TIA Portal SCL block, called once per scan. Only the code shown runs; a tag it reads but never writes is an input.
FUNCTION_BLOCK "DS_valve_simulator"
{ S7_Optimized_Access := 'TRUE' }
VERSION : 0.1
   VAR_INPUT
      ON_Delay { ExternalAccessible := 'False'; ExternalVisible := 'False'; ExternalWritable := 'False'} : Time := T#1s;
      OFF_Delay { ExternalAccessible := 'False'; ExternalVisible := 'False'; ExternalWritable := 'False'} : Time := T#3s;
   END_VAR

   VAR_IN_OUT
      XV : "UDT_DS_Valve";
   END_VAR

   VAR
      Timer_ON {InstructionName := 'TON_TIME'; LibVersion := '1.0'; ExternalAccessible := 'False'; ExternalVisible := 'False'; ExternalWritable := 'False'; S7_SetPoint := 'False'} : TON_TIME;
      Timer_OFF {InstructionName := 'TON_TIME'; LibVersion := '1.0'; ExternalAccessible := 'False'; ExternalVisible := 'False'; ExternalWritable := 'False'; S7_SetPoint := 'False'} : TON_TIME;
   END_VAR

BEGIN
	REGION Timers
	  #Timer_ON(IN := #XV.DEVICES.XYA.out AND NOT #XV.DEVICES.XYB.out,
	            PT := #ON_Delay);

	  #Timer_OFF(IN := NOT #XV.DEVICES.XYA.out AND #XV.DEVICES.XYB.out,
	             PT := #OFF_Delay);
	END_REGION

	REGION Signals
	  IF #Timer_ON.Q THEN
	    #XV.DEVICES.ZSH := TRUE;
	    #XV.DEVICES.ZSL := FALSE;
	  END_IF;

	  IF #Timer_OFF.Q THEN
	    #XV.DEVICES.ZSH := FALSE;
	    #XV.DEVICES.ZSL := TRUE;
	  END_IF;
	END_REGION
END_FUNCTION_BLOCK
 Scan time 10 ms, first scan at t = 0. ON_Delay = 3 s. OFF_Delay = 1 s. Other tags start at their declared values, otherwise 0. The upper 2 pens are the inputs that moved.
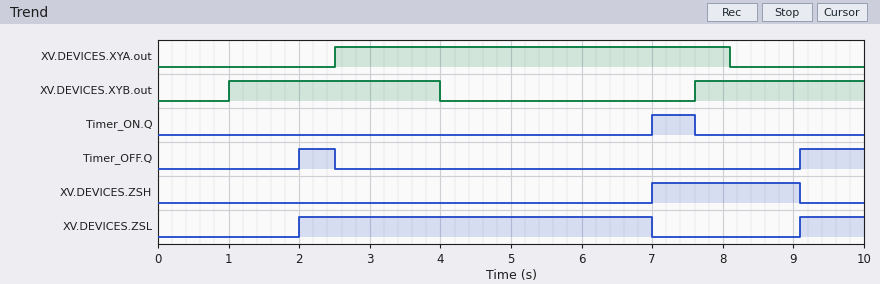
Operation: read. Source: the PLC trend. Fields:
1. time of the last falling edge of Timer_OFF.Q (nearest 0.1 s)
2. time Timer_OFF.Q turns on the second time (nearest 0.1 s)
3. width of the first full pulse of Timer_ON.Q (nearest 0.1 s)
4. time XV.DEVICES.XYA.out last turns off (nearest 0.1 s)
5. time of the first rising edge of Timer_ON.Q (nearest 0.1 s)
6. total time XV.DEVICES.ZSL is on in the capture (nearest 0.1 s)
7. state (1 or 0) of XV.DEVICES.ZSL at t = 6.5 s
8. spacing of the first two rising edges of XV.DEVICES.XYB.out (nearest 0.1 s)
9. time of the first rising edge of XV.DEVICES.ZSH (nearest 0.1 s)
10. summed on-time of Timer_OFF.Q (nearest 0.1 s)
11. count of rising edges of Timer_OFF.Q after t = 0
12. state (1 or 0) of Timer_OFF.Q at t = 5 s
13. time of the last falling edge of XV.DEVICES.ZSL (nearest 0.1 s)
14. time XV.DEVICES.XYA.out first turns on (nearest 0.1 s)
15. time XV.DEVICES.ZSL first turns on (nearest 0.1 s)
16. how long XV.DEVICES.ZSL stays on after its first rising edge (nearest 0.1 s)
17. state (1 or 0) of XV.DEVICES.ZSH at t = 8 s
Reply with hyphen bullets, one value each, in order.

- 2.5 s
- 9.1 s
- 0.6 s
- 8.1 s
- 7.0 s
- 5.9 s
- 1
- 6.6 s
- 7.0 s
- 1.4 s
- 2
- 0
- 7.0 s
- 2.5 s
- 2.0 s
- 5.0 s
- 1
